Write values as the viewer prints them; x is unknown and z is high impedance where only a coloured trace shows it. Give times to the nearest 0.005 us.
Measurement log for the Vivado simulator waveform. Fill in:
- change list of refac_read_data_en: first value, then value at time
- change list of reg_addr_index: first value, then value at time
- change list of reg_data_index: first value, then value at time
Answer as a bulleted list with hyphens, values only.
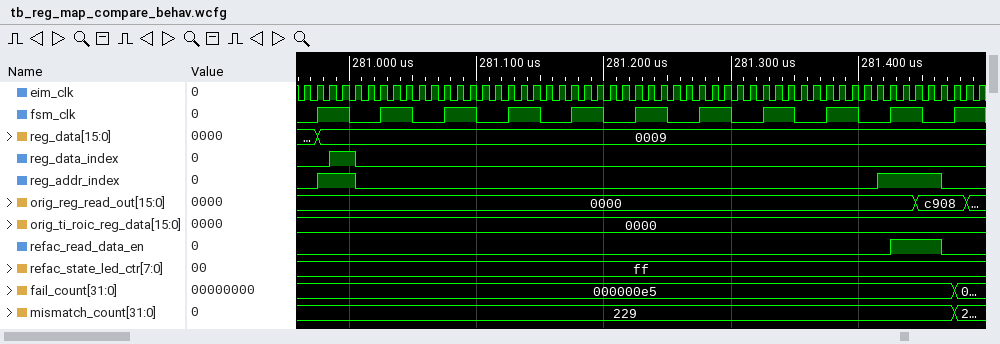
- 0, 1 at 281.425 us, 0 at 281.465 us
- 0, 1 at 280.975 us, 0 at 281.005 us, 1 at 281.415 us, 0 at 281.465 us
- 0, 1 at 280.985 us, 0 at 281.005 us
